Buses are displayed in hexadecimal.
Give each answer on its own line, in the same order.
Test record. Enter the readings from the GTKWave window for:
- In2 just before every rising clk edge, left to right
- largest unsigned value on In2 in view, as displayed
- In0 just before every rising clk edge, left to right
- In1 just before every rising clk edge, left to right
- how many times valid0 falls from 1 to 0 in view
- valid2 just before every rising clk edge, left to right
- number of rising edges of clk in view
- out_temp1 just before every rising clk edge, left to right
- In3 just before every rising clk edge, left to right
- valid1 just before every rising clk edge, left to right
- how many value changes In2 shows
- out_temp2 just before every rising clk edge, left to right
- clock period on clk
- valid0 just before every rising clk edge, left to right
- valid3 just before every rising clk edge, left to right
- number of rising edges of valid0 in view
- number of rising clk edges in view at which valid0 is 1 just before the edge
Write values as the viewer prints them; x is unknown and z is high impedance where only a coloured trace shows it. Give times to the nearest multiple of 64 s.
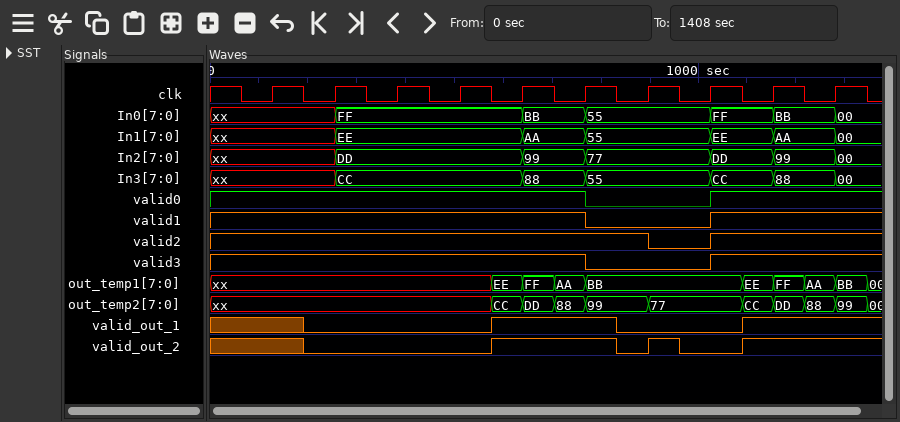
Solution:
xx, xx, DD, DD, DD, 99, 77, 77, DD, 99
DD
xx, xx, FF, FF, FF, BB, 55, 55, FF, BB
xx, xx, EE, EE, EE, AA, 55, 55, EE, AA
1
1 1 1 1 1 1 1 0 1 1
10
xx, xx, xx, xx, EE, AA, BB, BB, EE, AA
xx, xx, CC, CC, CC, 88, 55, 55, CC, 88
1 1 1 1 1 1 0 0 1 1
6
xx, xx, xx, xx, CC, 88, 99, 77, CC, 88
128 s
1 1 1 1 1 1 0 0 1 1
1 1 1 1 1 1 0 0 1 1
1
8
